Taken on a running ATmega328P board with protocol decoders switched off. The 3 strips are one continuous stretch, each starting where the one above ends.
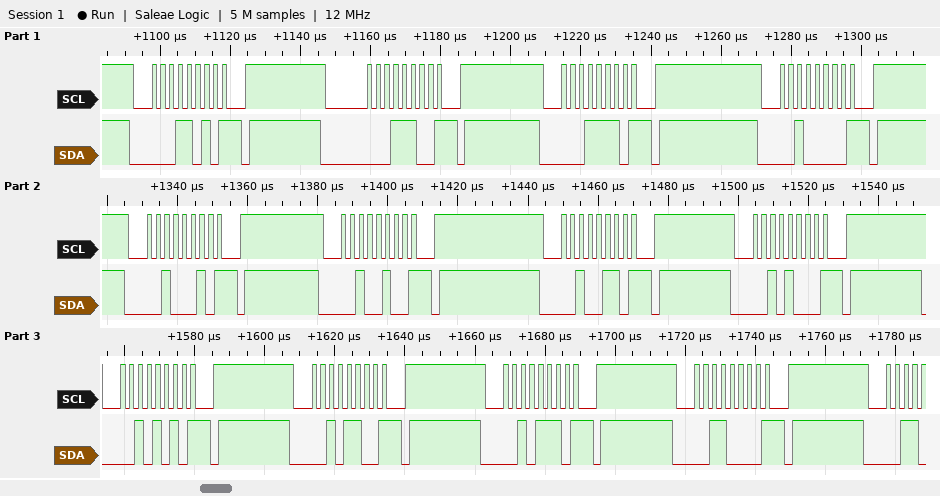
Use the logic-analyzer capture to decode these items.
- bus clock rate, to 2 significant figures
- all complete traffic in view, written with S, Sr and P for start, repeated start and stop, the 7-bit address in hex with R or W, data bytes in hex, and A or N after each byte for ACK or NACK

400 kHz
S 0DW N P S 0EW N P S 0FW N P S 10W N P S 11W N P S 12W N P S 13W N P S 14W N P S 15W N P S 16W N P S 17W N P S 18W N P
